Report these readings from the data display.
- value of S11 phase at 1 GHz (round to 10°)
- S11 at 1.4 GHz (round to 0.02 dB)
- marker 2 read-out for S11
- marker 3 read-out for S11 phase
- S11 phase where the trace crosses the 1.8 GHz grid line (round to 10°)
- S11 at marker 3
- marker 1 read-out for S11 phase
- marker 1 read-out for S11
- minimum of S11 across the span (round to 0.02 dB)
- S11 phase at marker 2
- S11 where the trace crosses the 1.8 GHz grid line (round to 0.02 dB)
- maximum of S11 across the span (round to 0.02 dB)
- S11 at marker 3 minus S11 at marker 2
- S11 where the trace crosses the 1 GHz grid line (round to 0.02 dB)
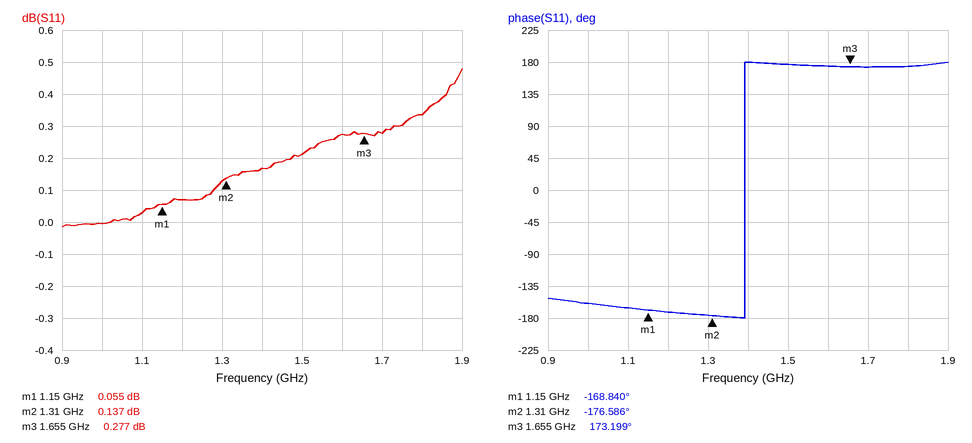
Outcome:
-160°
0.16 dB
0.137 dB
173.199°
170°
0.277 dB
-168.840°
0.055 dB
-0.02 dB
-176.586°
0.34 dB
0.48 dB
0.140 dB
0.00 dB
